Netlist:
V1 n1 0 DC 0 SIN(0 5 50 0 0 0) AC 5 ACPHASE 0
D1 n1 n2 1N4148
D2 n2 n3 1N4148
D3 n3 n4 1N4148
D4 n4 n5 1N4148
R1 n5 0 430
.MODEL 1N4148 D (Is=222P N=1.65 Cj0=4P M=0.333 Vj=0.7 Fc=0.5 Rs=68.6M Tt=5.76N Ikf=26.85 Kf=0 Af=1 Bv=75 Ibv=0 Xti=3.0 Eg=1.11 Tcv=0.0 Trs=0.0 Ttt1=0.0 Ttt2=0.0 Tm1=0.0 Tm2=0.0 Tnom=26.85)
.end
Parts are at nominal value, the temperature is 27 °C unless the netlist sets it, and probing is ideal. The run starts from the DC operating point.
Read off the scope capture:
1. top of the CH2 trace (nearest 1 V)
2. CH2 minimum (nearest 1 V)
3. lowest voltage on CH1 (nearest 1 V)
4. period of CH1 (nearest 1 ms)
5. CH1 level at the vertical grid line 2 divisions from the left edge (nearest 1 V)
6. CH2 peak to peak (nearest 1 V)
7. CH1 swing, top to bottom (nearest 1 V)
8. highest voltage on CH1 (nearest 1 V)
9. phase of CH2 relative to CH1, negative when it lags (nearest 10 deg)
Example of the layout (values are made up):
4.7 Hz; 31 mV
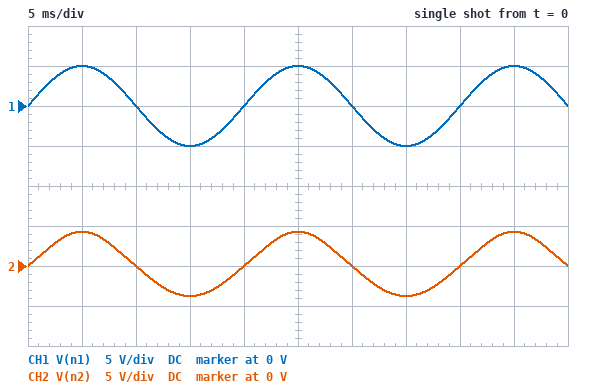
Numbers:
4 V; -4 V; -5 V; 20 ms; 0 V; 8 V; 10 V; 5 V; 0 deg
